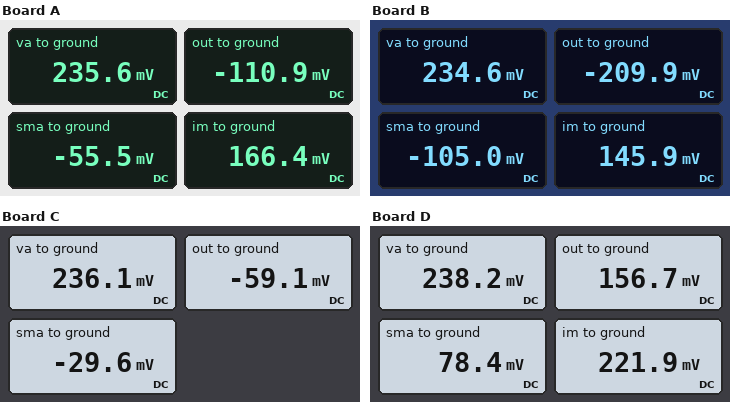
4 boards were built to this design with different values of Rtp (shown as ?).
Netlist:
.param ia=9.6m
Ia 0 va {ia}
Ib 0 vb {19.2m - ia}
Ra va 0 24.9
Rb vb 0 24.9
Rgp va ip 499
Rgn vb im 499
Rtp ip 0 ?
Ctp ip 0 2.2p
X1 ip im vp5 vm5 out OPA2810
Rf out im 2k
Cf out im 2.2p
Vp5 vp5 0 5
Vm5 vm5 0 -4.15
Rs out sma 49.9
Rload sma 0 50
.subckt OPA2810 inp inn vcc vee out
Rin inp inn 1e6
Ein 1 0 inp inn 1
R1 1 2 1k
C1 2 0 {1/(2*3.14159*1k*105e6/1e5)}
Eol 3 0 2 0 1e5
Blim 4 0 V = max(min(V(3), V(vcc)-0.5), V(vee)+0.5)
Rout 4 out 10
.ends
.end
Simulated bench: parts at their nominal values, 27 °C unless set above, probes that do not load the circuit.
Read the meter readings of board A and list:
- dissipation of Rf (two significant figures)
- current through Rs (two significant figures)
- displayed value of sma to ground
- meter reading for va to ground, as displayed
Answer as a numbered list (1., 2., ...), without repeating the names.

1. 38 µW
2. 1.1 mA
3. -55.5 mV
4. 235.6 mV
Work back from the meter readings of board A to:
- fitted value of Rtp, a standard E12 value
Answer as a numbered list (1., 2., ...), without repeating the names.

1. 1.2 kΩ
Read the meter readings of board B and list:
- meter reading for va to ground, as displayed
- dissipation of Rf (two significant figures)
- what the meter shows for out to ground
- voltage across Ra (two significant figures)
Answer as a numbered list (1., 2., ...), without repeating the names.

1. 234.6 mV
2. 63 µW
3. -209.9 mV
4. 230 mV
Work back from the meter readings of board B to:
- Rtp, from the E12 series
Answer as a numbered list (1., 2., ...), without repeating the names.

1. 820 Ω
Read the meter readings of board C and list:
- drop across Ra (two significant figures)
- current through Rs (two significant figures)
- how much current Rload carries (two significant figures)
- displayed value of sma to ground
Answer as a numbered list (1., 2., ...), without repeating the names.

1. 240 mV
2. 590 µA
3. 590 µA
4. -29.6 mV
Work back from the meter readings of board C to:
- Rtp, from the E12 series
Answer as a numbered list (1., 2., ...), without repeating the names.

1. 1.5 kΩ
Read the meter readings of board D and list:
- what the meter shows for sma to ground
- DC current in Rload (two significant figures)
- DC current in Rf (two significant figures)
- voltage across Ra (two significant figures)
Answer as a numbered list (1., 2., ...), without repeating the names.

1. 78.4 mV
2. 1.6 mA
3. 33 µA
4. 240 mV
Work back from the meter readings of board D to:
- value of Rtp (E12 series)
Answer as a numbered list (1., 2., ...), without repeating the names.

1. 6.8 kΩ
